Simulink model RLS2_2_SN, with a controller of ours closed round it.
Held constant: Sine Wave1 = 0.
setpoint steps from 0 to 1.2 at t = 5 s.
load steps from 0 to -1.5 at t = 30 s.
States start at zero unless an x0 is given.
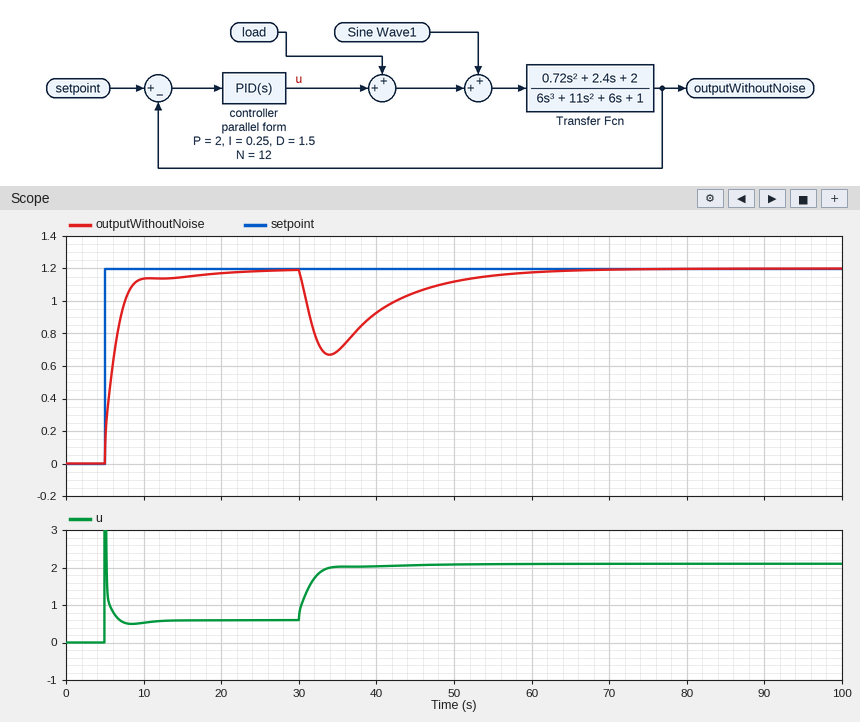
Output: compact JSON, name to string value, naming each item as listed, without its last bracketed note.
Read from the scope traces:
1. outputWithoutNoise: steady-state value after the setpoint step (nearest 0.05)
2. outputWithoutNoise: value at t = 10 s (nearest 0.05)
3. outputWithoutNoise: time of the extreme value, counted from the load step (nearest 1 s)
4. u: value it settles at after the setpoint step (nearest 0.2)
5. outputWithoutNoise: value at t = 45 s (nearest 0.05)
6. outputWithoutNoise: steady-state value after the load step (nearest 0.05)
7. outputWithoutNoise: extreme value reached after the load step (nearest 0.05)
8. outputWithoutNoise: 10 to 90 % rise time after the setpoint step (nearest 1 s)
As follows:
{"outputWithoutNoise: steady-state value after the setpoint step": "1.20", "outputWithoutNoise: value at t = 10 s": "1.15", "outputWithoutNoise: time of the extreme value, counted from the load step": "4 s", "u: value it settles at after the setpoint step": "0.6", "outputWithoutNoise: value at t = 45 s": "1.05", "outputWithoutNoise: steady-state value after the load step": "1.20", "outputWithoutNoise: extreme value reached after the load step": "0.65", "outputWithoutNoise: 10 to 90 % rise time after the setpoint step": "3 s"}
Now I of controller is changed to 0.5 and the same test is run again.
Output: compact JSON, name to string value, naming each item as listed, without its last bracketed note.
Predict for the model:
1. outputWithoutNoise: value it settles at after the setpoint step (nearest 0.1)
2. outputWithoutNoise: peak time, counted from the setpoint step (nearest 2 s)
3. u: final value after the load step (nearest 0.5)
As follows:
{"outputWithoutNoise: value it settles at after the setpoint step": "1.2", "outputWithoutNoise: peak time, counted from the setpoint step": "6 s", "u: final value after the load step": "2.0"}
